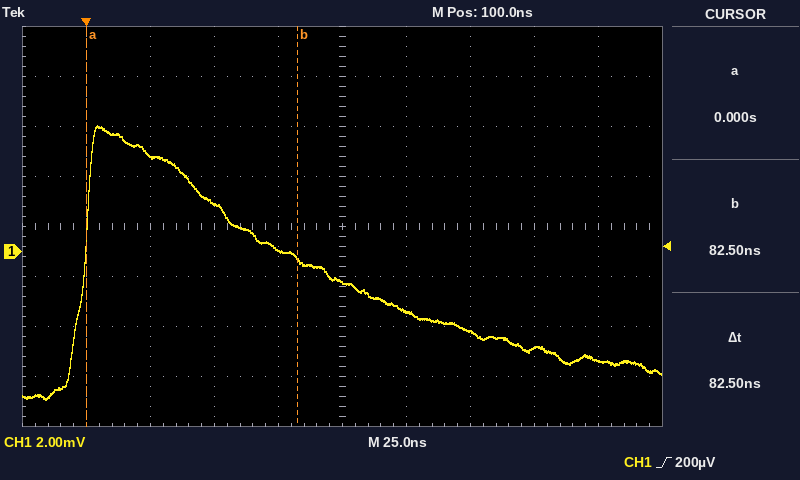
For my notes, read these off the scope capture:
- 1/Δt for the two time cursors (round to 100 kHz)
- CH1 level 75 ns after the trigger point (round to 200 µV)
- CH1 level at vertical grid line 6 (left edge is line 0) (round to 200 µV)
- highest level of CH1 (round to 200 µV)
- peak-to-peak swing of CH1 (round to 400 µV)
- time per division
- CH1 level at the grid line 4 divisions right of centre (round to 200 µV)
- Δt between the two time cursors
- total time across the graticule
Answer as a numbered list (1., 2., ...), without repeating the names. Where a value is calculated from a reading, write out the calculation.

1. 1 / 82.5 ns ≈ 12.1 MHz
2. 0.0 mV
3. -2.4 mV
4. 5.0 mV
5. 10.8 mV
6. 25 ns
7. -4.4 mV
8. 82.5 ns
9. 250 ns
